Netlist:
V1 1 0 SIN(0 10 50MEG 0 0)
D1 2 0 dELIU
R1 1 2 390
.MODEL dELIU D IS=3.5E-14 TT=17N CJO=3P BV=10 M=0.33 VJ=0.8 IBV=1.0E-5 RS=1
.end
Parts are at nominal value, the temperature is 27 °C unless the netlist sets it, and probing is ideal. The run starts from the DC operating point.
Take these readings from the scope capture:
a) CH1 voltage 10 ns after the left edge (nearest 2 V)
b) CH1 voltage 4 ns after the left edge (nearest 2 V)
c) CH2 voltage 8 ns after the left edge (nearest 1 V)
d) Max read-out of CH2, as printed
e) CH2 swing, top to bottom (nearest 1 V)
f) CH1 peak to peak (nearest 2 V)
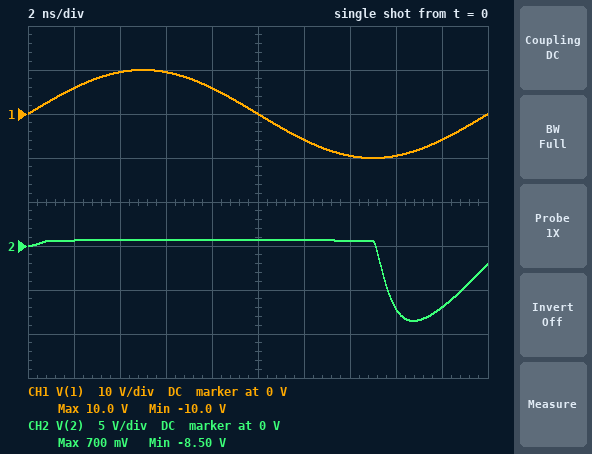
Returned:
0 V
10 V
1 V
700 mV
9 V
20 V
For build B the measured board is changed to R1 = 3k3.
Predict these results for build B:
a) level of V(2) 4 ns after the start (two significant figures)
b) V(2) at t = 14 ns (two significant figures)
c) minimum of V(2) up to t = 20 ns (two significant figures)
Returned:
590 mV
570 mV
-2.6 V
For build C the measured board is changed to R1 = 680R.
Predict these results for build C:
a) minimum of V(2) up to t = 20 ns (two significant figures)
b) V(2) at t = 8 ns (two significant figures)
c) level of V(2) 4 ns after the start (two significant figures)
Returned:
-7.4 V
660 mV
650 mV
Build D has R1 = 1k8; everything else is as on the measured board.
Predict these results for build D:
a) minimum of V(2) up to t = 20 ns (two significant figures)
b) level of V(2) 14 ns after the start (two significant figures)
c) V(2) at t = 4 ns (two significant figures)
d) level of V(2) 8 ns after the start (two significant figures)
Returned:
-4.4 V
590 mV
610 mV
630 mV
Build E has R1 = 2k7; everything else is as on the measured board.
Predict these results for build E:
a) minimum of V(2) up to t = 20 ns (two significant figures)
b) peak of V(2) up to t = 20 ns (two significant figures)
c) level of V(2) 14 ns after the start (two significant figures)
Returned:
-3.2 V
620 mV
580 mV
